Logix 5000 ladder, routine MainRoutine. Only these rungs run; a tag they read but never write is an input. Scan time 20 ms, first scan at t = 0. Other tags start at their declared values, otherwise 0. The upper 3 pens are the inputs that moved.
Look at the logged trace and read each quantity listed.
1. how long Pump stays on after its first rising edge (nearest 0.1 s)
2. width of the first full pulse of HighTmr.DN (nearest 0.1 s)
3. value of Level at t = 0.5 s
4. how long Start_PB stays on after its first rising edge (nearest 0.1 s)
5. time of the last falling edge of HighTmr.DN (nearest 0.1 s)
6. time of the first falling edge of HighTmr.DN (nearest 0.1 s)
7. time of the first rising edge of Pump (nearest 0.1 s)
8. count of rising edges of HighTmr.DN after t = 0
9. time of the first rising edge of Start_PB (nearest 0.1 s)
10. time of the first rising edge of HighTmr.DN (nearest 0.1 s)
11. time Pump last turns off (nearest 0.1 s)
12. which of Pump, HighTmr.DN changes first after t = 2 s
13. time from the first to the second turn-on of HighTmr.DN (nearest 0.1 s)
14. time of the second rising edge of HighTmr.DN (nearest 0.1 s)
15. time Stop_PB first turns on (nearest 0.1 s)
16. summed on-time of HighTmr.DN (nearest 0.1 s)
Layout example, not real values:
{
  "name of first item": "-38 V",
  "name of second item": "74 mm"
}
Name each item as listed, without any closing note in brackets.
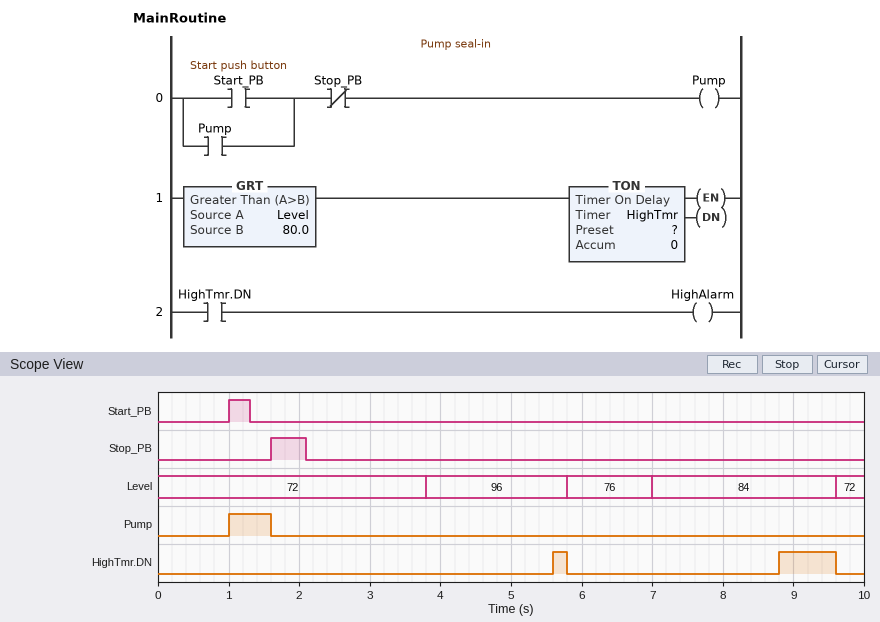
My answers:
{
  "how long Pump stays on after its first rising edge": "0.6 s",
  "width of the first full pulse of HighTmr.DN": "0.2 s",
  "value of Level at t = 0.5 s": "72",
  "how long Start_PB stays on after its first rising edge": "0.3 s",
  "time of the last falling edge of HighTmr.DN": "9.6 s",
  "time of the first falling edge of HighTmr.DN": "5.8 s",
  "time of the first rising edge of Pump": "1.0 s",
  "count of rising edges of HighTmr.DN after t = 0": "2",
  "time of the first rising edge of Start_PB": "1.0 s",
  "time of the first rising edge of HighTmr.DN": "5.6 s",
  "time Pump last turns off": "1.6 s",
  "which of Pump, HighTmr.DN changes first after t = 2 s": "HighTmr.DN",
  "time from the first to the second turn-on of HighTmr.DN": "3.2 s",
  "time of the second rising edge of HighTmr.DN": "8.8 s",
  "time Stop_PB first turns on": "1.6 s",
  "summed on-time of HighTmr.DN": "1.0 s"
}
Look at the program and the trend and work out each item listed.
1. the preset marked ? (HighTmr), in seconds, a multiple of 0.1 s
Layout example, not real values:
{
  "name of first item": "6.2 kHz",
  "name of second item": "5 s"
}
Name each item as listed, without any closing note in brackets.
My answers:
{
  "the preset marked ? (HighTmr), in seconds, a multiple of 0.1 s": "1.8 s"
}
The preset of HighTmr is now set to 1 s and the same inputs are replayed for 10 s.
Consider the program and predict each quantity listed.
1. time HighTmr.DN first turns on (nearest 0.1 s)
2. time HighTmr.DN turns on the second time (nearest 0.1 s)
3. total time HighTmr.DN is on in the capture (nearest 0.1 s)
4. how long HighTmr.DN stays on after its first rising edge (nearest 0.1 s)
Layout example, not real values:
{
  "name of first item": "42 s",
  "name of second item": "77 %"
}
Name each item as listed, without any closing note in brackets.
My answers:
{
  "time HighTmr.DN first turns on": "4.8 s",
  "time HighTmr.DN turns on the second time": "8.0 s",
  "total time HighTmr.DN is on in the capture": "2.6 s",
  "how long HighTmr.DN stays on after its first rising edge": "1.0 s"
}
